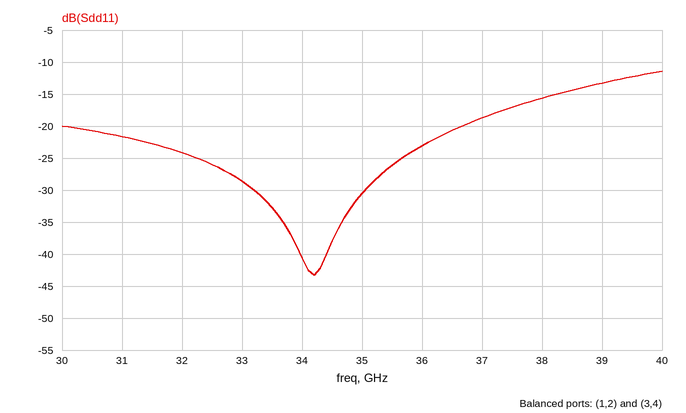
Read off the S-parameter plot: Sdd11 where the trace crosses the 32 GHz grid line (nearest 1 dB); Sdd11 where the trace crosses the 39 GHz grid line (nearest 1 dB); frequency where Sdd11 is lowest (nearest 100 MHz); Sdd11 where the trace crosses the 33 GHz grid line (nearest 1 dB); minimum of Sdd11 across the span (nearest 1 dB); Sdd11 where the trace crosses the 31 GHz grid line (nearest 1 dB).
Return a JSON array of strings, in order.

["-24 dB", "-13 dB", "34.2 GHz", "-29 dB", "-43 dB", "-22 dB"]
